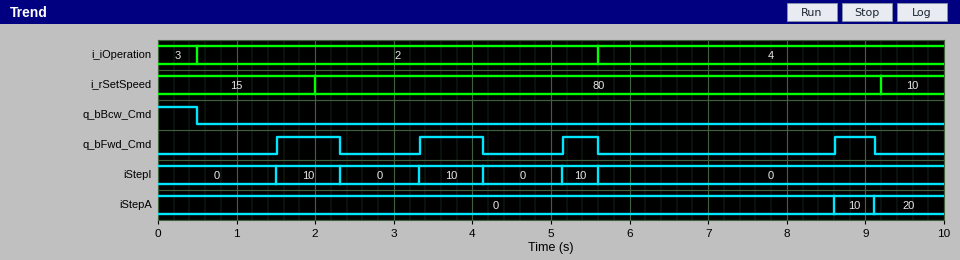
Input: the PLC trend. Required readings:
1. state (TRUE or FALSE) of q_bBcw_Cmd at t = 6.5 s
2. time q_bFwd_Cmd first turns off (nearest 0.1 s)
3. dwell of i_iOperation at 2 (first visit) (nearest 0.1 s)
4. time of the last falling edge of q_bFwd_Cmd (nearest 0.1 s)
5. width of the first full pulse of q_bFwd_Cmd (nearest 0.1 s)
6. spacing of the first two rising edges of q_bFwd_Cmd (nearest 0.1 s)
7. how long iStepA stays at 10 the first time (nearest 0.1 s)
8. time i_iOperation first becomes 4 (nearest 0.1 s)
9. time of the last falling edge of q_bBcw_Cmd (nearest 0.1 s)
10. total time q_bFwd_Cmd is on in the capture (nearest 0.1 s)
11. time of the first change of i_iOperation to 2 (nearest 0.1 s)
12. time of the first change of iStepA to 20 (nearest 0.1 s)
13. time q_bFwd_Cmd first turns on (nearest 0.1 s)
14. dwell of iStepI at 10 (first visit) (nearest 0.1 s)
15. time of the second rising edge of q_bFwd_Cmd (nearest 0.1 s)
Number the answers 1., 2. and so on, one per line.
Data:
1. FALSE
2. 2.3 s
3. 5.1 s
4. 9.1 s
5. 0.8 s
6. 1.8 s
7. 0.5 s
8. 5.6 s
9. 0.5 s
10. 2.6 s
11. 0.5 s
12. 9.1 s
13. 1.5 s
14. 0.8 s
15. 3.3 s
